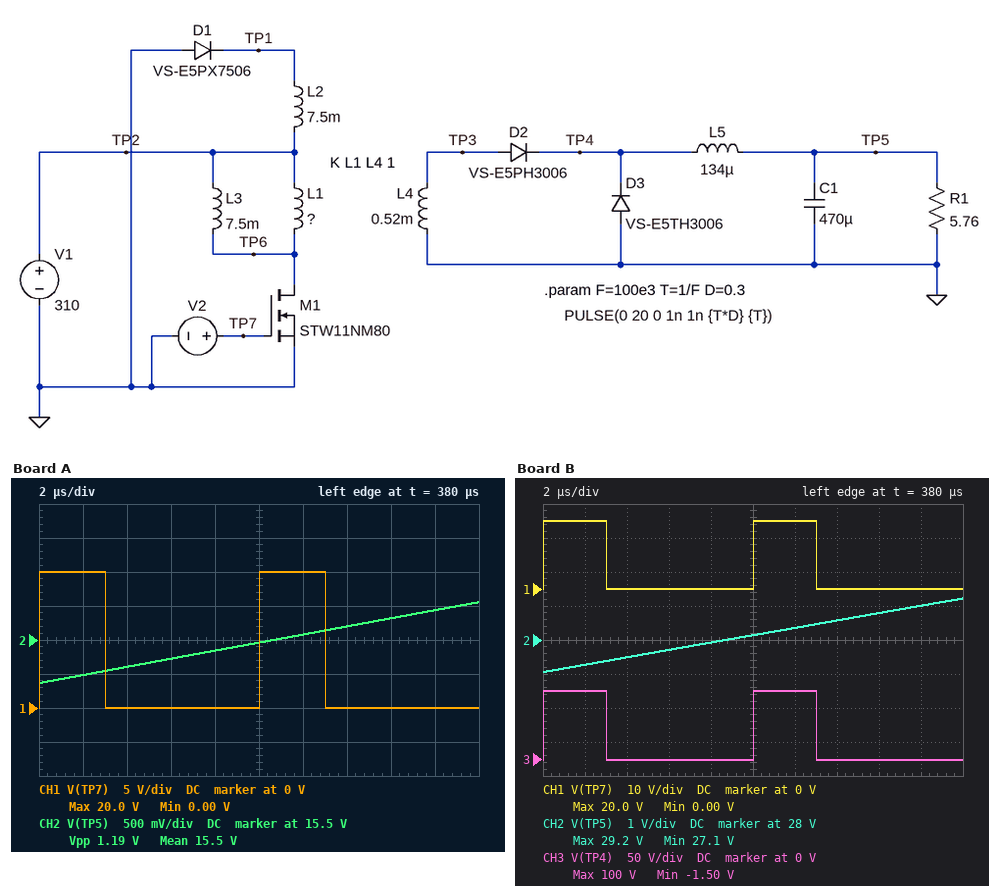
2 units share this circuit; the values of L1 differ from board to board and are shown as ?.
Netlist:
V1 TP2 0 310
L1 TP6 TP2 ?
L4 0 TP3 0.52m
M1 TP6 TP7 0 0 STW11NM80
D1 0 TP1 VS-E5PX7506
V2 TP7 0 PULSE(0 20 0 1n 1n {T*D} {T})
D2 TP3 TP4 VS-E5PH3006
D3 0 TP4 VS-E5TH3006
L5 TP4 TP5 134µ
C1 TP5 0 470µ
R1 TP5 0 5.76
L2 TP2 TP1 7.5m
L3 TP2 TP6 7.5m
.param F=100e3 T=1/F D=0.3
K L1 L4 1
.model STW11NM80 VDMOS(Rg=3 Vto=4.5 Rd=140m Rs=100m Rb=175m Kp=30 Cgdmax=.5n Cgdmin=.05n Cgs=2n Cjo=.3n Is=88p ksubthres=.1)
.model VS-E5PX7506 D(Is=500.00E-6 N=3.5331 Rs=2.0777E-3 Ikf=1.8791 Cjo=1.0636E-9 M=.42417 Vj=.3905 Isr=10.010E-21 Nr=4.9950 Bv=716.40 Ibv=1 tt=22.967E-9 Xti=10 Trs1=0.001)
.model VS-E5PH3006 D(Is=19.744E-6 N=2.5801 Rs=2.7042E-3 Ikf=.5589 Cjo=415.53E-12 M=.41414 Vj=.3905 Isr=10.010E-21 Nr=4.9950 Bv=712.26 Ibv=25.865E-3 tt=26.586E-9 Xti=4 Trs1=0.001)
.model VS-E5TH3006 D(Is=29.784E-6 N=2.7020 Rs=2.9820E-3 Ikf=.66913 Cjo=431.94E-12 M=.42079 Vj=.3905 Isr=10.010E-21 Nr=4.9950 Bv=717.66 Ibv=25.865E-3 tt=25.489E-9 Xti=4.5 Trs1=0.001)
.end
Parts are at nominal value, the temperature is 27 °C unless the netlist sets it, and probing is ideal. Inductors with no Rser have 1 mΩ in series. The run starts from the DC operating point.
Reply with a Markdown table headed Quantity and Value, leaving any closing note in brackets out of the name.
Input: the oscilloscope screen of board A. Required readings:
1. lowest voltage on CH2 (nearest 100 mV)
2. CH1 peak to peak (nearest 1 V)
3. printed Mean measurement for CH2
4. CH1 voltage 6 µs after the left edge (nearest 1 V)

| Quantity | Value |
|---|---|
| lowest voltage on CH2 | 14.9 V |
| CH1 peak to peak | 20 V |
| printed Mean measurement for CH2 | 15.5 V |
| CH1 voltage 6 µs after the left edge | 0 V |
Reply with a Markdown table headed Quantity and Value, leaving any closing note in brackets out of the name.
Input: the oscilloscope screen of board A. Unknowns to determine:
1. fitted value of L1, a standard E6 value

| Quantity | Value |
|---|---|
| fitted value of L1, a standard E6 value | 15 mH |
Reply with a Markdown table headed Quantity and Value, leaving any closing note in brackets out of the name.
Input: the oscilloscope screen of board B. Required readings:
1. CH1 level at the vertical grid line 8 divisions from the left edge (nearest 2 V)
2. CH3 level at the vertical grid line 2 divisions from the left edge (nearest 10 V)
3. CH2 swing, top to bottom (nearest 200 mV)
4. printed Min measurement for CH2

| Quantity | Value |
|---|---|
| CH1 level at the vertical grid line 8 divisions from the left edge | 0 V |
| CH3 level at the vertical grid line 2 divisions from the left edge | 0 V |
| CH2 swing, top to bottom | 2.2 V |
| printed Min measurement for CH2 | 27.1 V |
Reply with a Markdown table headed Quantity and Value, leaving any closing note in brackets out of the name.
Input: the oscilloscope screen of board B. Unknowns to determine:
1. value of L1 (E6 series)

| Quantity | Value |
|---|---|
| value of L1 | 4.7 mH |
